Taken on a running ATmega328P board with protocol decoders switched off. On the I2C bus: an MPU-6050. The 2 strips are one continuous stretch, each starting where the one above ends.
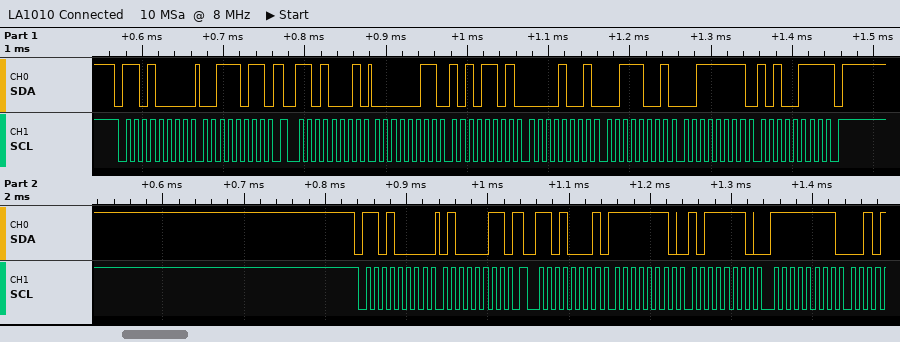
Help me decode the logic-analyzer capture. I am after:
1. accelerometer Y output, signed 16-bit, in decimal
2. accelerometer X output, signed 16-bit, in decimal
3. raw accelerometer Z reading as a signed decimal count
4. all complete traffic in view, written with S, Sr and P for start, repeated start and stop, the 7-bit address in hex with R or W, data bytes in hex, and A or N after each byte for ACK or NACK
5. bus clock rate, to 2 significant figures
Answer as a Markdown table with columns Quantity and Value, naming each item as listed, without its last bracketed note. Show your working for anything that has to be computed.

| Quantity | Value |
|---|---|
| accelerometer Y output, signed 16-bit, in decimal | 0x0939 = 2361 |
| accelerometer X output, signed 16-bit, in decimal | 0x03AD = 941 |
| raw accelerometer Z reading as a signed decimal count | 0x3FA7 = 16295 |
| all complete traffic in view, written with S, Sr and P for start, repeated start and stop, the 7-bit address in hex with R or W, data bytes in hex, and A or N after each byte for ACK or NACK | S 68W A 3B A Sr 68R A 03 A AD A 09 A 39 A 3F A A7 N P S 68W A 43 A Sr 68R A FE A BE A FF A |
| bus clock rate, to 2 significant figures | 100 kHz |
